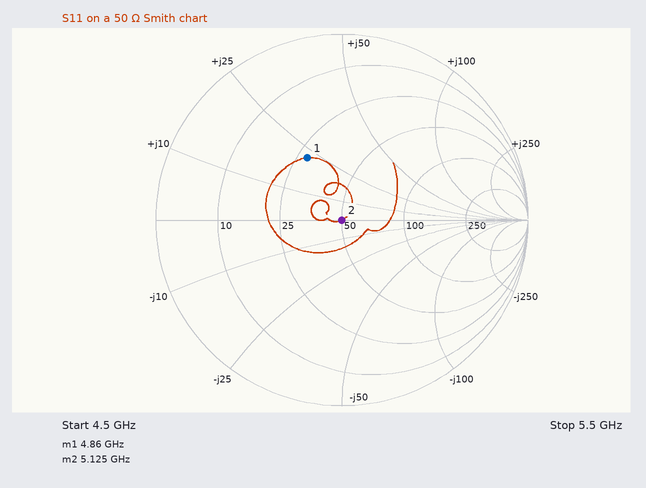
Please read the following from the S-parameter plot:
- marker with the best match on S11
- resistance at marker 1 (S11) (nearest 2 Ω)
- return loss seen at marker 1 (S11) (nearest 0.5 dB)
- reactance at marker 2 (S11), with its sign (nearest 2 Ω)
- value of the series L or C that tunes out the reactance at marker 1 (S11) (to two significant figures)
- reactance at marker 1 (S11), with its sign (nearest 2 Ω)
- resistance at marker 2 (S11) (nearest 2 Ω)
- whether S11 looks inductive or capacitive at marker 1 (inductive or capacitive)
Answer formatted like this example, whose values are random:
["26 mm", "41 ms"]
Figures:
["marker 2", "28 Ω", "8.5 dB", "0 Ω", "1.5 pF", "+22 Ω", "50 Ω", "inductive"]
